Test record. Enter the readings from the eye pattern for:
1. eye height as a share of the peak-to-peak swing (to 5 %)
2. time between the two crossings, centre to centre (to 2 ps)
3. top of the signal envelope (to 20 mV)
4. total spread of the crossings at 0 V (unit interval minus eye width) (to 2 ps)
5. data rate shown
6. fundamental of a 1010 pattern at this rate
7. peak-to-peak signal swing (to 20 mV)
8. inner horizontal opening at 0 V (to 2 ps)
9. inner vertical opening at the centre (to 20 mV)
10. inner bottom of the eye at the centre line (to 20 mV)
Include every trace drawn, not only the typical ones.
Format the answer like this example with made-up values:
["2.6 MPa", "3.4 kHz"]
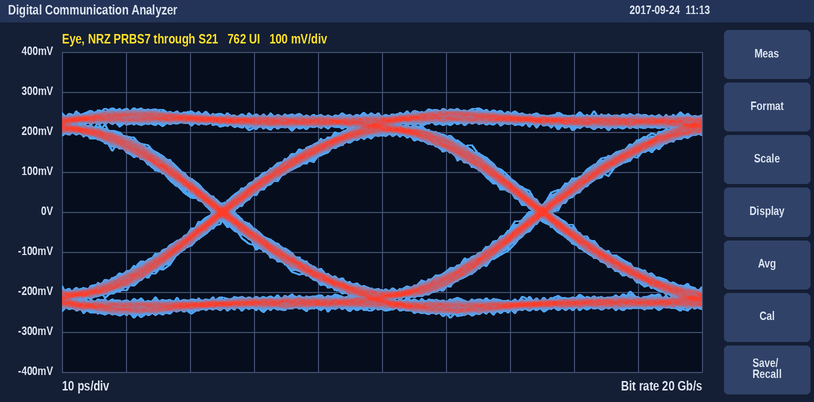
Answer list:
["75 %", "50 ps", "260 mV", "4 ps", "20 Gb/s", "10 GHz", "520 mV", "46 ps", "380 mV", "-200 mV"]
